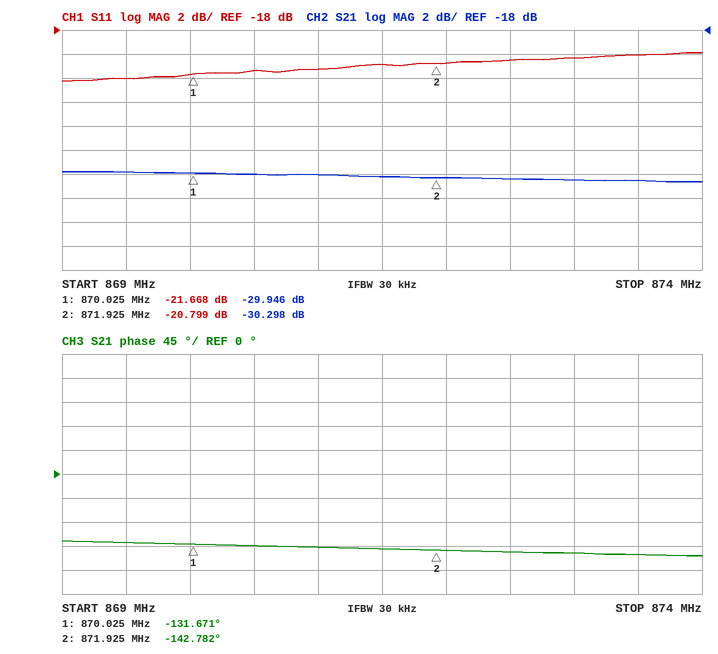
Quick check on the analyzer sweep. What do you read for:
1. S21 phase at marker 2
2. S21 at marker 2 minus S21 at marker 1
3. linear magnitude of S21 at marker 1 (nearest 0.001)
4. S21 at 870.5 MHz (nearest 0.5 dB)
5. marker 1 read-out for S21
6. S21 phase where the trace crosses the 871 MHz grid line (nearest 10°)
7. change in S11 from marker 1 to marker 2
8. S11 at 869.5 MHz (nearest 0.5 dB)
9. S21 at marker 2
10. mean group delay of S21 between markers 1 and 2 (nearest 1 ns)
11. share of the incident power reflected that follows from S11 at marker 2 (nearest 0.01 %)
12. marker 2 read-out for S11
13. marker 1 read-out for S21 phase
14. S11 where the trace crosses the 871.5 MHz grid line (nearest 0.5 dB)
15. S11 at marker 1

-142.782°
-0.352 dB
0.032
-30.0 dB
-29.946 dB
-140°
0.869 dB
-22.0 dB
-30.298 dB
16 ns
0.83 %
-20.799 dB
-131.671°
-21.0 dB
-21.668 dB
